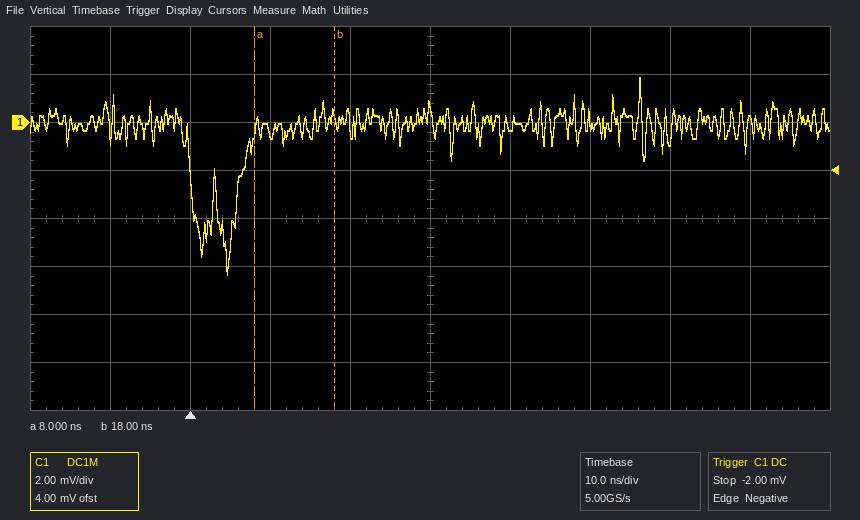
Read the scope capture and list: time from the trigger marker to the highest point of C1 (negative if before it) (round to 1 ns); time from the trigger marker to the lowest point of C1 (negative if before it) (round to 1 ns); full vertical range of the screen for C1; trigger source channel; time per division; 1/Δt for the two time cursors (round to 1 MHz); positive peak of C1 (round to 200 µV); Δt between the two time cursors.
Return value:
+56 ns
+5 ns
16 mV
C1
10 ns
100 MHz
1.8 mV
10 ns
